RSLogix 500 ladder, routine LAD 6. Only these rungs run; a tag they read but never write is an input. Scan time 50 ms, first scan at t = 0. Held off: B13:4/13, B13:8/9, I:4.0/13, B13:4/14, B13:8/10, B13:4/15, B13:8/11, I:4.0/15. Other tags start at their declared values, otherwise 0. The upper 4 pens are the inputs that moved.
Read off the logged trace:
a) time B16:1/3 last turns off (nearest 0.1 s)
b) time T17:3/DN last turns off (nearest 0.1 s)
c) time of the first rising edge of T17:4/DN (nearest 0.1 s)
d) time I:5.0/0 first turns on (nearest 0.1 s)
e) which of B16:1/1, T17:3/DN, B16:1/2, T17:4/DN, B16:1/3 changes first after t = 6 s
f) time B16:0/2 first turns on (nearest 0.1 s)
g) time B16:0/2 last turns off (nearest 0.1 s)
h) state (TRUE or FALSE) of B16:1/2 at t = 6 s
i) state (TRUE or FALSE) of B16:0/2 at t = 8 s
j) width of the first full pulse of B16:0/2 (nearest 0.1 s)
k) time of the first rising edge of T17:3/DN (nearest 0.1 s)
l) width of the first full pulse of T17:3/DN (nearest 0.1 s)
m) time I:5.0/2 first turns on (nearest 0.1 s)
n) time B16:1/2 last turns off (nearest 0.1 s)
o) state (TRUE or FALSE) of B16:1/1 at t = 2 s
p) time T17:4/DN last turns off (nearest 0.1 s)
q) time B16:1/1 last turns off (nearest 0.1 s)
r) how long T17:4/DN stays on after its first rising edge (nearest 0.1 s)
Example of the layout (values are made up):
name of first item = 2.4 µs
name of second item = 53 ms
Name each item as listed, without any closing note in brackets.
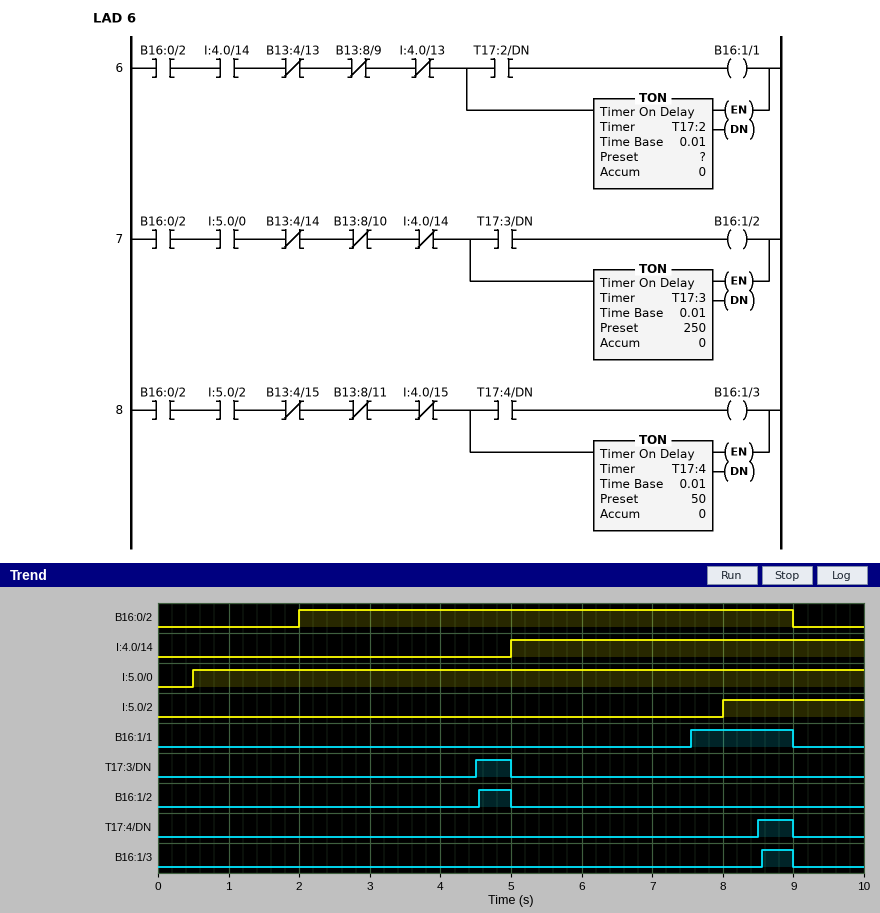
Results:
time B16:1/3 last turns off = 9.0 s
time T17:3/DN last turns off = 5.0 s
time of the first rising edge of T17:4/DN = 8.5 s
time I:5.0/0 first turns on = 0.5 s
which of B16:1/1, T17:3/DN, B16:1/2, T17:4/DN, B16:1/3 changes first after t = 6 s = B16:1/1
time B16:0/2 first turns on = 2.0 s
time B16:0/2 last turns off = 9.0 s
state (TRUE or FALSE) of B16:1/2 at t = 6 s = FALSE
state (TRUE or FALSE) of B16:0/2 at t = 8 s = TRUE
width of the first full pulse of B16:0/2 = 7.0 s
time of the first rising edge of T17:3/DN = 4.5 s
width of the first full pulse of T17:3/DN = 0.5 s
time I:5.0/2 first turns on = 8.0 s
time B16:1/2 last turns off = 5.0 s
state (TRUE or FALSE) of B16:1/1 at t = 2 s = FALSE
time T17:4/DN last turns off = 9.0 s
time B16:1/1 last turns off = 9.0 s
how long T17:4/DN stays on after its first rising edge = 0.5 s
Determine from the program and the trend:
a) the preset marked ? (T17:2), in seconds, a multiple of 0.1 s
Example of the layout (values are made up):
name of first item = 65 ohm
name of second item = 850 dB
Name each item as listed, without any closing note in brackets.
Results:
the preset marked ? (T17:2), in seconds, a multiple of 0.1 s = 2.5 s
